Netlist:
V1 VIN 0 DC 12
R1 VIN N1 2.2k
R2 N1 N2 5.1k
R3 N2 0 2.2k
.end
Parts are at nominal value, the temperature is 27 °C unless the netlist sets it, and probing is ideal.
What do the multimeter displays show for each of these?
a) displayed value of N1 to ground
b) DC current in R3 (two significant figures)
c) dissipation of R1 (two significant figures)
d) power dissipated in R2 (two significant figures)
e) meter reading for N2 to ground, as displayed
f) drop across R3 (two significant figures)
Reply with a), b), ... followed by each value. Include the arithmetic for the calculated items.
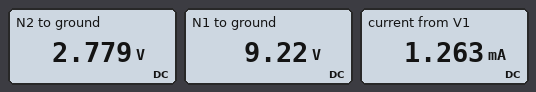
a) 9.22 V
b) (2.779 V) / 2.2 kΩ = 1.3 mA
c) (12 V - 9.22 V)^2 / 2.2 kΩ = 3.5 mW
d) (9.22 V - 2.779 V)^2 / 5.1 kΩ = 8.1 mW
e) 2.779 V
f) 2.779 V = 2.8 V
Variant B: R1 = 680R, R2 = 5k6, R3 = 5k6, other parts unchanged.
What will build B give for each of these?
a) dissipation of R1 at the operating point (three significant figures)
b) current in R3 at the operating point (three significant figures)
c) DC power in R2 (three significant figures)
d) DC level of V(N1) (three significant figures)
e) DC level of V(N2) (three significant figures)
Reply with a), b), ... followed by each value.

a) 694 µW
b) 1.01 mA
c) 5.71 mW
d) 11.3 V
e) 5.66 V
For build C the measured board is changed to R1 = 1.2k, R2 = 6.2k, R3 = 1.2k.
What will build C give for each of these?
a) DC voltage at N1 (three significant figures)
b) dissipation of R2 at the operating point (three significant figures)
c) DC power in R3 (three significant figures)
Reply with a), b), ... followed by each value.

a) 10.3 V
b) 12.1 mW
c) 2.34 mW
